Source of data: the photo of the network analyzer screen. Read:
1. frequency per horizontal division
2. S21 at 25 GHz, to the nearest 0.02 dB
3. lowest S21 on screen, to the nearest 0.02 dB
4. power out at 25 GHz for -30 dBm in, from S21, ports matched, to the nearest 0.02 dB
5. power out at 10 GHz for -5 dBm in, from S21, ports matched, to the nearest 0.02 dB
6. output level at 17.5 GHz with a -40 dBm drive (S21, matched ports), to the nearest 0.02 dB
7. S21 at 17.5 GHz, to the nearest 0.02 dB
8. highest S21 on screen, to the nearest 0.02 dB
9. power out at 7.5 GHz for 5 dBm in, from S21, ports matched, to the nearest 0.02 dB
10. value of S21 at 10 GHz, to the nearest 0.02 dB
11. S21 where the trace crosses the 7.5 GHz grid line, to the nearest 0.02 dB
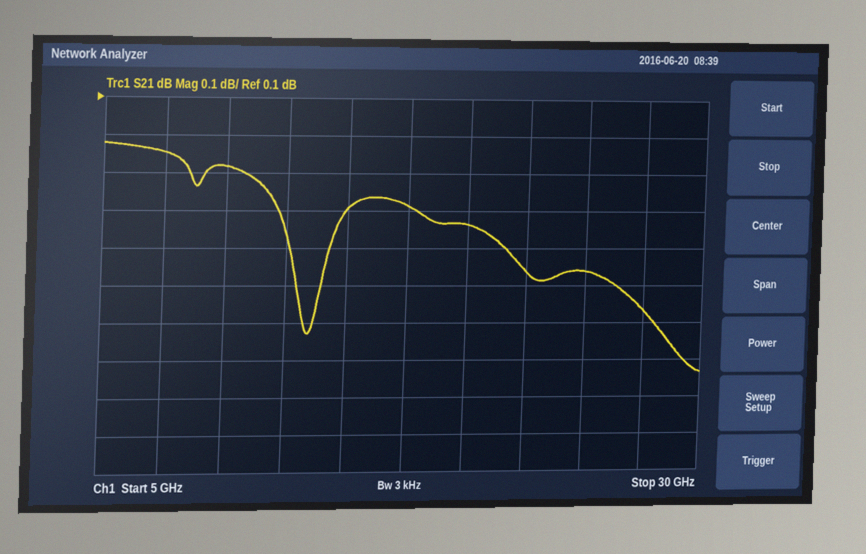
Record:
2.5 GHz
-0.36 dB
-0.64 dB
-30.36 dBm
-5.08 dBm
-40.18 dBm
-0.18 dB
-0.02 dB
4.96 dBm
-0.08 dB
-0.04 dB
